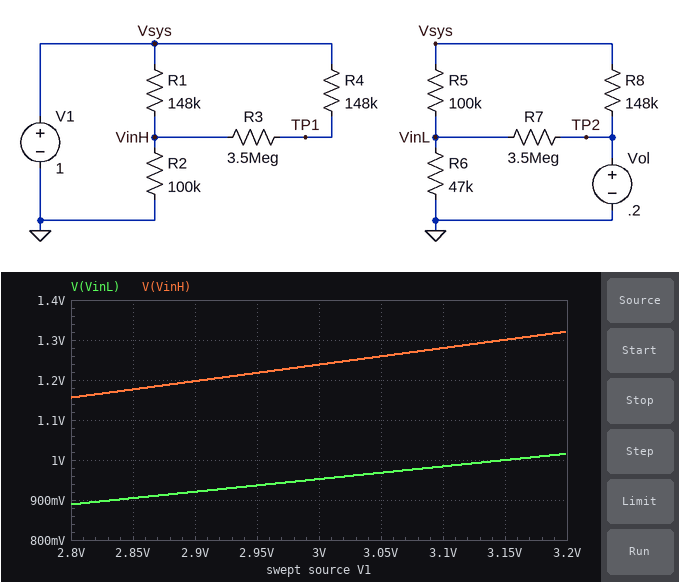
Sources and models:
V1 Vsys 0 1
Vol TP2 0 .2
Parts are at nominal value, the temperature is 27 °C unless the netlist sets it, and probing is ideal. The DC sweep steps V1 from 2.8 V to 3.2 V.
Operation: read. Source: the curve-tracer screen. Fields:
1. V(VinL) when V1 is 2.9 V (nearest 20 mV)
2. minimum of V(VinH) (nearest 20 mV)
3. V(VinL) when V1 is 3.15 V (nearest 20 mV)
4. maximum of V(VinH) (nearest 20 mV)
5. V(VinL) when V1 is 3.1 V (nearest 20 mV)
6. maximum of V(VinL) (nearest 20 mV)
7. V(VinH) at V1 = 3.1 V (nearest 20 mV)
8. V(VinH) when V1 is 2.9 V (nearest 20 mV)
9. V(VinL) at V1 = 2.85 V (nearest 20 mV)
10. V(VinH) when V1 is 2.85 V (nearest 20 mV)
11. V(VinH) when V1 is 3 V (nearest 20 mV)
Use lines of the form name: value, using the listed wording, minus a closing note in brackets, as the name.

V(VinL) when V1 is 2.9 V: 920 mV
minimum of V(VinH): 1.16 V
V(VinL) when V1 is 3.15 V: 1.00 V
maximum of V(VinH): 1.32 V
V(VinL) when V1 is 3.1 V: 980 mV
maximum of V(VinL): 1.02 V
V(VinH) at V1 = 3.1 V: 1.28 V
V(VinH) when V1 is 2.9 V: 1.20 V
V(VinL) at V1 = 2.85 V: 900 mV
V(VinH) when V1 is 2.85 V: 1.18 V
V(VinH) when V1 is 3 V: 1.24 V
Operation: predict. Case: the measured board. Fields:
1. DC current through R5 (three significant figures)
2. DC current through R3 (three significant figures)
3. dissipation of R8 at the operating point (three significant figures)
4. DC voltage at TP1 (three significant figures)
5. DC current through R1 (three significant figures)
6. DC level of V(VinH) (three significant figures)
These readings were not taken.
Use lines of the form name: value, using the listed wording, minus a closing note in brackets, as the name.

DC current through R5: 6.81 µA
DC current through R3: 161 nA
dissipation of R8 at the operating point: 4.32 µW
DC voltage at TP1: 976 mV
DC current through R1: 3.97 µA
DC level of V(VinH): 413 mV
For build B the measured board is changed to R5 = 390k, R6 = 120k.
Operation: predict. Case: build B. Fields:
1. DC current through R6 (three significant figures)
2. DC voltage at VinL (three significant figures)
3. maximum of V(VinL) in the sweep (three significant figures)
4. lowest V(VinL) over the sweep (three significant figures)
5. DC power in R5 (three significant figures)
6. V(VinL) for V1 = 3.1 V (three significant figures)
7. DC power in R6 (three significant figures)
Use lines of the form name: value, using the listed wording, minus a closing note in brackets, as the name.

DC current through R6: 1.95 µA
DC voltage at VinL: 234 mV
maximum of V(VinL) in the sweep: 739 mV
lowest V(VinL) over the sweep: 647 mV
DC power in R5: 1.50 µW
V(VinL) for V1 = 3.1 V: 716 mV
DC power in R6: 458 nW
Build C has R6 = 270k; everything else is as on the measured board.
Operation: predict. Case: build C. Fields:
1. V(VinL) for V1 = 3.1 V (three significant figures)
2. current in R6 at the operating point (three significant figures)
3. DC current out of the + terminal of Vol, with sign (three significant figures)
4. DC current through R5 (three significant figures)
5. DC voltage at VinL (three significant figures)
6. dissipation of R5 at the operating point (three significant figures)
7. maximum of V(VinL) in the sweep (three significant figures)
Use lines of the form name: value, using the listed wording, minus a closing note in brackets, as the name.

V(VinL) for V1 = 3.1 V: 2.22 V
current in R6 at the operating point: 2.66 µA
DC current out of the + terminal of Vol, with sign: -5.55 µA
DC current through R5: 2.81 µA
DC voltage at VinL: 719 mV
dissipation of R5 at the operating point: 790 nW
maximum of V(VinL) in the sweep: 2.29 V
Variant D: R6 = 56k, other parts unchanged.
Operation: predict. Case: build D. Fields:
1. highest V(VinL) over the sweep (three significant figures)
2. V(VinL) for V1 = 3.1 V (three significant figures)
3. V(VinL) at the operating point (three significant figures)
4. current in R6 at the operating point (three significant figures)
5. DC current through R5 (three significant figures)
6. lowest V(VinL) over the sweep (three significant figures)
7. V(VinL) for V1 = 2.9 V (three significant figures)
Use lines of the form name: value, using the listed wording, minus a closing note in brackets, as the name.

highest V(VinL) over the sweep: 1.14 V
V(VinL) for V1 = 3.1 V: 1.10 V
V(VinL) at the operating point: 357 mV
current in R6 at the operating point: 6.38 µA
DC current through R5: 6.43 µA
lowest V(VinL) over the sweep: 997 mV
V(VinL) for V1 = 2.9 V: 1.03 V
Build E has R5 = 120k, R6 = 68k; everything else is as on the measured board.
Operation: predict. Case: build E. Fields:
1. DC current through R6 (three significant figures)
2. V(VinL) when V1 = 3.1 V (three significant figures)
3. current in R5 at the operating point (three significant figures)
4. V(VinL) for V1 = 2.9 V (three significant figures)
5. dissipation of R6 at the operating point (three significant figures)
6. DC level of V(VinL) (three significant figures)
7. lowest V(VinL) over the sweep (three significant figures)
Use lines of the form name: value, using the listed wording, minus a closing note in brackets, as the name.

DC current through R6: 5.29 µA
V(VinL) when V1 = 3.1 V: 1.11 V
current in R5 at the operating point: 5.34 µA
V(VinL) for V1 = 2.9 V: 1.04 V
dissipation of R6 at the operating point: 1.90 µW
DC level of V(VinL): 360 mV
lowest V(VinL) over the sweep: 1.00 V
